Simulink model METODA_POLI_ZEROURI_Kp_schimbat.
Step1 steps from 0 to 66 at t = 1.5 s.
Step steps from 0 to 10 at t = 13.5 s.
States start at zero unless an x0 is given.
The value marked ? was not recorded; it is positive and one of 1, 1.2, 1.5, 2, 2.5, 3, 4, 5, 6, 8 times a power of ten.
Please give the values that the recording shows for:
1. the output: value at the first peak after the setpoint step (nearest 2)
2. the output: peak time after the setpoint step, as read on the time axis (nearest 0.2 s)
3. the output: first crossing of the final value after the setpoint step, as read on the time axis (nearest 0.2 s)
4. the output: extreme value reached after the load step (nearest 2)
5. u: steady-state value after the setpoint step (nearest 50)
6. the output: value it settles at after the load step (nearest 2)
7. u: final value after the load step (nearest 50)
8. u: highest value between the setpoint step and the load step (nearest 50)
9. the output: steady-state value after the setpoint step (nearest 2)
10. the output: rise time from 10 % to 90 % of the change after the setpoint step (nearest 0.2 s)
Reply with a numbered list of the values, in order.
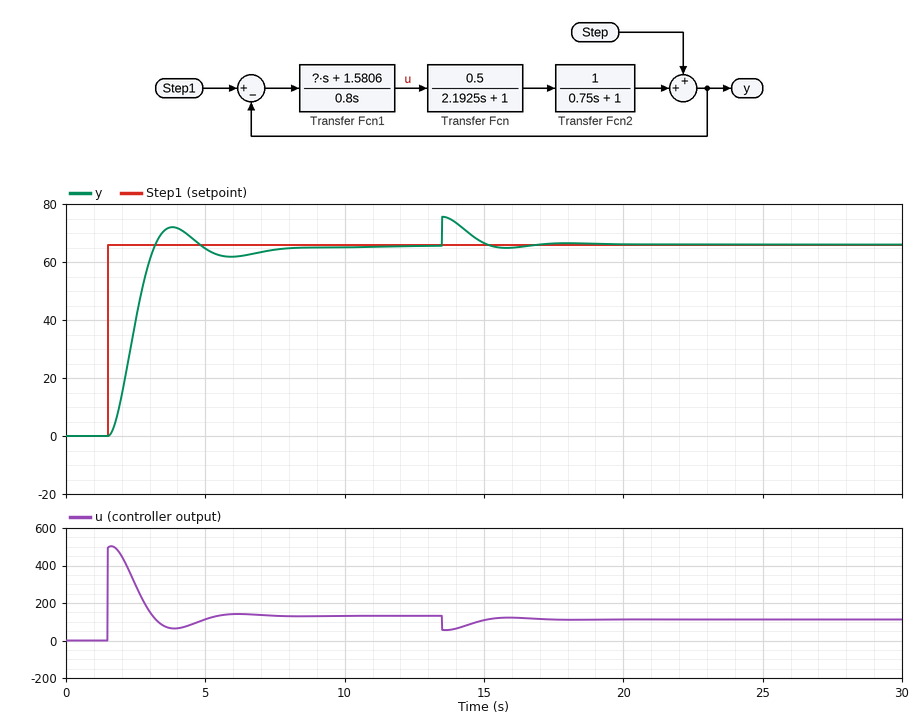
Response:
1. 72
2. 3.8 s
3. 3.2 s
4. 76
5. 150
6. 66
7. 100
8. 500
9. 66
10. 1.2 s
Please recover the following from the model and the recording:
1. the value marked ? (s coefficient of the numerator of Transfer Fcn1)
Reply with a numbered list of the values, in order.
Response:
1. 6
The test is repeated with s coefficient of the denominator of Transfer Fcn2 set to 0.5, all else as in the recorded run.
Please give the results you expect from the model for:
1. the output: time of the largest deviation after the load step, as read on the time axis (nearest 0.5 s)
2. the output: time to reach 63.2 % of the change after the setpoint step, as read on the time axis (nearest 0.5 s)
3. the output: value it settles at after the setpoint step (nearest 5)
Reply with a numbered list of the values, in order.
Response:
1. 13.5 s
2. 2.5 s
3. 65
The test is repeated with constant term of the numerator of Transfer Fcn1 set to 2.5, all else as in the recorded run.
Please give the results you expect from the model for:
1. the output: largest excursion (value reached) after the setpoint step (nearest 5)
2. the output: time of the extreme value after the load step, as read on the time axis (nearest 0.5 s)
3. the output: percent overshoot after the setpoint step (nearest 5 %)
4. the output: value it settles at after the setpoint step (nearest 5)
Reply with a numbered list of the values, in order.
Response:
1. 80
2. 13.5 s
3. 20 %
4. 65
